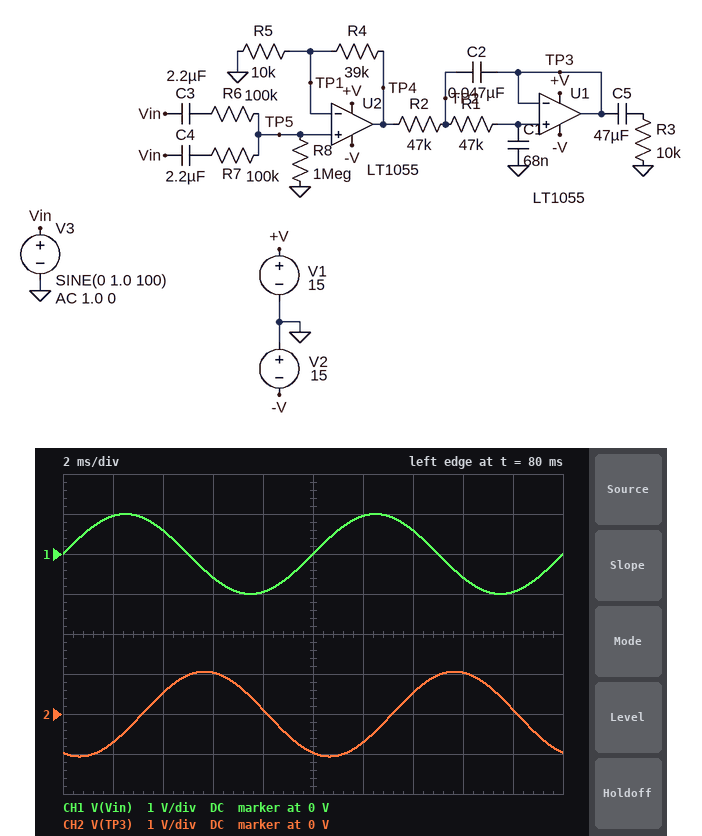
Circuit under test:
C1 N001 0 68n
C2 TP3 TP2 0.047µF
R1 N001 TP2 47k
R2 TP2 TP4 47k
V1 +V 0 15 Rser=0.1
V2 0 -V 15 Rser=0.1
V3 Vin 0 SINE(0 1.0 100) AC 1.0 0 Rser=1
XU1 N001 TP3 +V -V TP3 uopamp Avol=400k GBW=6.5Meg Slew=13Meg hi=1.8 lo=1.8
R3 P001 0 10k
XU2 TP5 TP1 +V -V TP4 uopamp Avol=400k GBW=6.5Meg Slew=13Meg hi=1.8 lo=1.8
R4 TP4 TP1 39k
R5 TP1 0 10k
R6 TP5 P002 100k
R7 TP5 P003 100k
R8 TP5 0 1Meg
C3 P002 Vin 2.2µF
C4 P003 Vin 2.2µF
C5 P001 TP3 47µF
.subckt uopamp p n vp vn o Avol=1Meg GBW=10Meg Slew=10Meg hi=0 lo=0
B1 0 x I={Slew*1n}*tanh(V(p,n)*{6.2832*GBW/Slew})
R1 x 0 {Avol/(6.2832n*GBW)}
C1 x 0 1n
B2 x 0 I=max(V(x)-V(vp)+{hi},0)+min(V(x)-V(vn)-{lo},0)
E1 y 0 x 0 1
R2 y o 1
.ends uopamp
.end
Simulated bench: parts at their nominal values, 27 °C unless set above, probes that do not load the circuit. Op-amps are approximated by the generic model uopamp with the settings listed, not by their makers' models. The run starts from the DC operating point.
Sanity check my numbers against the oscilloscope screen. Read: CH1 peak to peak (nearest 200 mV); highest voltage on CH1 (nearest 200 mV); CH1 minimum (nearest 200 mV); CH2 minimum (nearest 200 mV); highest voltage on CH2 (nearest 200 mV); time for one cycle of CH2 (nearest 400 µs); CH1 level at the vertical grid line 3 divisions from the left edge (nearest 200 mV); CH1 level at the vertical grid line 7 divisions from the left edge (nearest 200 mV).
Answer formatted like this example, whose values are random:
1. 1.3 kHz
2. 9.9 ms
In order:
1. 2.0 V
2. 1.0 V
3. -1.0 V
4. -1.0 V
5. 1.0 V
6. 10.0 ms
7. -600 mV
8. 600 mV
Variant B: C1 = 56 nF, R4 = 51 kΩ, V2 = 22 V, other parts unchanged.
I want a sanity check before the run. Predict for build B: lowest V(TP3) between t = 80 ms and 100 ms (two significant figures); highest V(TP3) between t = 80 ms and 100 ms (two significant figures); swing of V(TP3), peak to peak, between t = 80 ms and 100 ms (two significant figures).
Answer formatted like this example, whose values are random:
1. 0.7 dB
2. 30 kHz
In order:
1. -1.6 V
2. 1.6 V
3. 3.3 V
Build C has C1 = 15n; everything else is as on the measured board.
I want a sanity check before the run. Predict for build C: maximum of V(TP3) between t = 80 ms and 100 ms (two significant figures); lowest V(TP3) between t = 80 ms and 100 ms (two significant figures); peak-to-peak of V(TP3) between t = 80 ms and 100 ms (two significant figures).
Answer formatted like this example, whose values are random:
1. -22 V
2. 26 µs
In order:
1. 4.8 V
2. -4.8 V
3. 9.7 V
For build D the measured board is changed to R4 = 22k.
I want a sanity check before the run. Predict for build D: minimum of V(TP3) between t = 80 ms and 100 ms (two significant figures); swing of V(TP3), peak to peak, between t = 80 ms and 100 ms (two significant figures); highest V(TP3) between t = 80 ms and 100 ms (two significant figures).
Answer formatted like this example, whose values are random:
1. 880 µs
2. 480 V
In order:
1. -690 mV
2. 1.4 V
3. 690 mV
